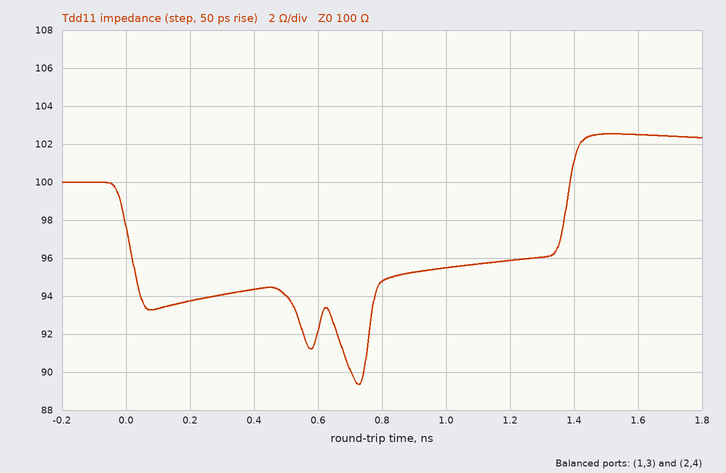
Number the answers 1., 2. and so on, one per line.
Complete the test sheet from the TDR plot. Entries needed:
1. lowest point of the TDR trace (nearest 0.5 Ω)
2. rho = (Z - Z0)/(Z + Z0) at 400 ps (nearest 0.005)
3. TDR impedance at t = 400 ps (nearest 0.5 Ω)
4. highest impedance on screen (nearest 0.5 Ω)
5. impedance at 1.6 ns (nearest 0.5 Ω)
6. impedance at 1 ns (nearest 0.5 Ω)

1. 89.5 Ω
2. -0.030
3. 94.5 Ω
4. 102.5 Ω
5. 102.5 Ω
6. 95.5 Ω
